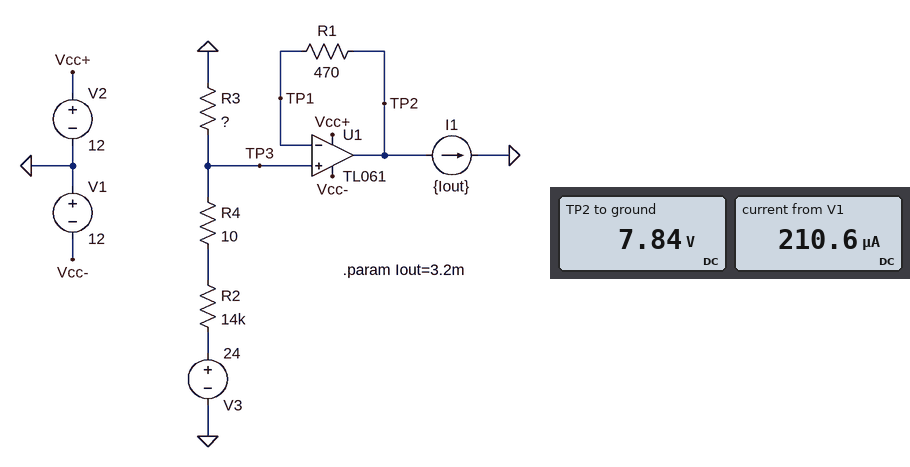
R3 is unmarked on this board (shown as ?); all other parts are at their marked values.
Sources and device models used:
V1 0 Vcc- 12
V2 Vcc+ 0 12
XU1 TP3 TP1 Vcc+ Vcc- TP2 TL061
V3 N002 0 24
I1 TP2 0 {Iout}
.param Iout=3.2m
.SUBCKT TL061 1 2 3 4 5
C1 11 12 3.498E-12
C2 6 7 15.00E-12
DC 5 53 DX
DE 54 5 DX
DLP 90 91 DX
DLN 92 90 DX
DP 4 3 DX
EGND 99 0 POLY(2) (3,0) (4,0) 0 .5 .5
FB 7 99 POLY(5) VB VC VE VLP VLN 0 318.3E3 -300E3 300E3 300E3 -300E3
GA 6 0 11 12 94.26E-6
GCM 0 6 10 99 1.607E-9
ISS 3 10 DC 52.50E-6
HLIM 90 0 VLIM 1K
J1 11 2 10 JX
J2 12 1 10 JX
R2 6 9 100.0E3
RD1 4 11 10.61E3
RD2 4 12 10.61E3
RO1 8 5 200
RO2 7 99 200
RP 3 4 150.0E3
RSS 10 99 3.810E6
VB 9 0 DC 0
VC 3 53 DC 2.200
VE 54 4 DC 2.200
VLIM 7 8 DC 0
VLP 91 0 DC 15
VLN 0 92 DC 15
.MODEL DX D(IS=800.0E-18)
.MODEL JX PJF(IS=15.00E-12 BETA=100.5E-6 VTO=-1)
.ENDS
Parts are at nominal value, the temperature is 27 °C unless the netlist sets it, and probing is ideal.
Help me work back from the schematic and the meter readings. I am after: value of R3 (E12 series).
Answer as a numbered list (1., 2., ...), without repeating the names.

1. 6.8 kΩ
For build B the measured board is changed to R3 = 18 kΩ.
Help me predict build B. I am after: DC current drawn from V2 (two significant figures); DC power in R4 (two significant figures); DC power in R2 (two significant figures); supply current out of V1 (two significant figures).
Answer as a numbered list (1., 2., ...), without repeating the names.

1. 160 µA
2. 5.6 µW
3. 7.9 mW
4. 210 µA
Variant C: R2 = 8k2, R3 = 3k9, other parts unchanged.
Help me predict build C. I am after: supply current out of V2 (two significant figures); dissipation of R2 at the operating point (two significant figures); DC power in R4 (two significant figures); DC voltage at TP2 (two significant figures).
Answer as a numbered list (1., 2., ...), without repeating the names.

1. 210 µA
2. 32 mW
3. 39 µW
4. 7.7 V
